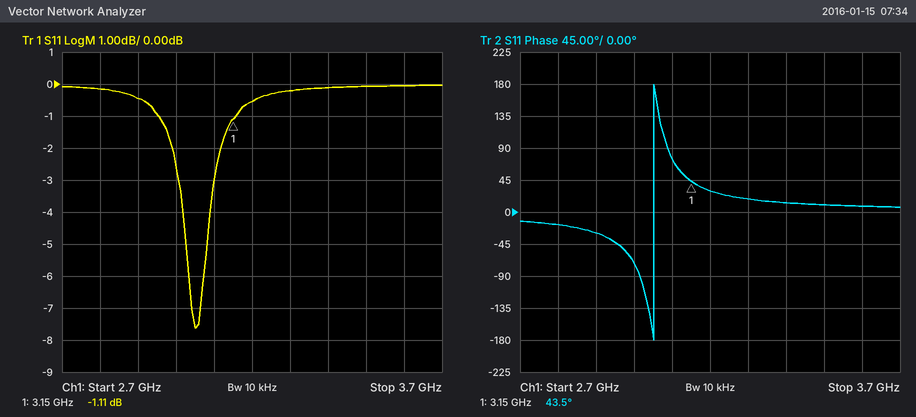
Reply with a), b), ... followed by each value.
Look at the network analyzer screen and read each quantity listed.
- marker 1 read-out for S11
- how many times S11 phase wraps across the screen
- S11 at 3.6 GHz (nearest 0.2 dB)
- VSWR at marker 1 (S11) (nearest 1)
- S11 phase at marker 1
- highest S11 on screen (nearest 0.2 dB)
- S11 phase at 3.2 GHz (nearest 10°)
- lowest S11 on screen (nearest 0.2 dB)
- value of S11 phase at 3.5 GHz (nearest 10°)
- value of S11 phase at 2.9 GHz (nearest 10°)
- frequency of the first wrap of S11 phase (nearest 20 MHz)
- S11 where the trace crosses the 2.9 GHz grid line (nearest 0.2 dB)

a) -1.11 dB
b) 1
c) 0.0 dB
d) 16
e) 43.5°
f) 0.0 dB
g) 30°
h) -7.6 dB
i) 10°
j) -30°
k) 3.06 GHz
l) -0.4 dB
